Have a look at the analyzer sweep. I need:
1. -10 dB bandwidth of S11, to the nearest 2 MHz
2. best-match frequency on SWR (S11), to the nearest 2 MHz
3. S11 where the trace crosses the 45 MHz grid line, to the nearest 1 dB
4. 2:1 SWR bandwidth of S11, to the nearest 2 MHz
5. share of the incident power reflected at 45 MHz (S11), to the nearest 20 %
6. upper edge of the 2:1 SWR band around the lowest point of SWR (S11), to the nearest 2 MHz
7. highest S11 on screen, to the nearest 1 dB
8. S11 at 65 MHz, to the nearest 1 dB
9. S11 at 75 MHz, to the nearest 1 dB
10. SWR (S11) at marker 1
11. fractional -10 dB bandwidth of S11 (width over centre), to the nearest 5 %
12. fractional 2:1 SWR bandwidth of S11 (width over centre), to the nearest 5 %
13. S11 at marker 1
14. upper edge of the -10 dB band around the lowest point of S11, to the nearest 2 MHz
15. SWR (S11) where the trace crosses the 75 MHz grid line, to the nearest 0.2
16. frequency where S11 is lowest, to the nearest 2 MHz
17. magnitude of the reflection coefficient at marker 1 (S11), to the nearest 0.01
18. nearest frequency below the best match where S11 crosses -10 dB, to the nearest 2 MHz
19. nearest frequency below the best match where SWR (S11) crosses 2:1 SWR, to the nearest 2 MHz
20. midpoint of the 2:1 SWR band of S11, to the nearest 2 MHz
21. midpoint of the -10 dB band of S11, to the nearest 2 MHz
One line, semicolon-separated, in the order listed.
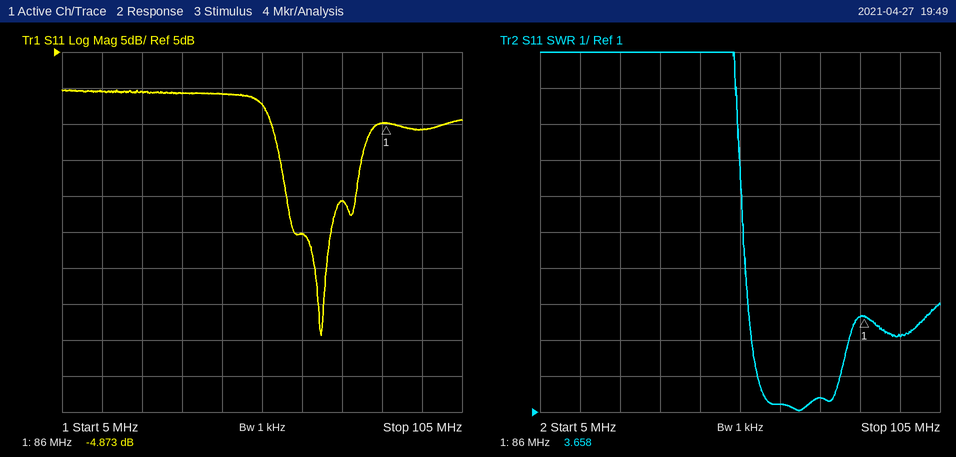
20 MHz; 70 MHz; -1 dB; 20 MHz; 80 %; 80 MHz; 0 dB; -20 dB; -16 dB; 3.658; 30 %; 30 %; -4.873 dB; 80 MHz; 1.4; 70 MHz; 0.57; 60 MHz; 60 MHz; 70 MHz; 70 MHz
